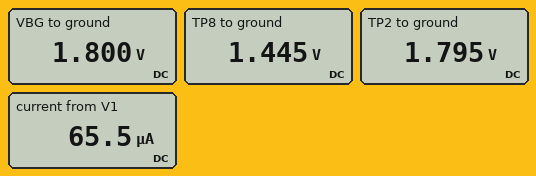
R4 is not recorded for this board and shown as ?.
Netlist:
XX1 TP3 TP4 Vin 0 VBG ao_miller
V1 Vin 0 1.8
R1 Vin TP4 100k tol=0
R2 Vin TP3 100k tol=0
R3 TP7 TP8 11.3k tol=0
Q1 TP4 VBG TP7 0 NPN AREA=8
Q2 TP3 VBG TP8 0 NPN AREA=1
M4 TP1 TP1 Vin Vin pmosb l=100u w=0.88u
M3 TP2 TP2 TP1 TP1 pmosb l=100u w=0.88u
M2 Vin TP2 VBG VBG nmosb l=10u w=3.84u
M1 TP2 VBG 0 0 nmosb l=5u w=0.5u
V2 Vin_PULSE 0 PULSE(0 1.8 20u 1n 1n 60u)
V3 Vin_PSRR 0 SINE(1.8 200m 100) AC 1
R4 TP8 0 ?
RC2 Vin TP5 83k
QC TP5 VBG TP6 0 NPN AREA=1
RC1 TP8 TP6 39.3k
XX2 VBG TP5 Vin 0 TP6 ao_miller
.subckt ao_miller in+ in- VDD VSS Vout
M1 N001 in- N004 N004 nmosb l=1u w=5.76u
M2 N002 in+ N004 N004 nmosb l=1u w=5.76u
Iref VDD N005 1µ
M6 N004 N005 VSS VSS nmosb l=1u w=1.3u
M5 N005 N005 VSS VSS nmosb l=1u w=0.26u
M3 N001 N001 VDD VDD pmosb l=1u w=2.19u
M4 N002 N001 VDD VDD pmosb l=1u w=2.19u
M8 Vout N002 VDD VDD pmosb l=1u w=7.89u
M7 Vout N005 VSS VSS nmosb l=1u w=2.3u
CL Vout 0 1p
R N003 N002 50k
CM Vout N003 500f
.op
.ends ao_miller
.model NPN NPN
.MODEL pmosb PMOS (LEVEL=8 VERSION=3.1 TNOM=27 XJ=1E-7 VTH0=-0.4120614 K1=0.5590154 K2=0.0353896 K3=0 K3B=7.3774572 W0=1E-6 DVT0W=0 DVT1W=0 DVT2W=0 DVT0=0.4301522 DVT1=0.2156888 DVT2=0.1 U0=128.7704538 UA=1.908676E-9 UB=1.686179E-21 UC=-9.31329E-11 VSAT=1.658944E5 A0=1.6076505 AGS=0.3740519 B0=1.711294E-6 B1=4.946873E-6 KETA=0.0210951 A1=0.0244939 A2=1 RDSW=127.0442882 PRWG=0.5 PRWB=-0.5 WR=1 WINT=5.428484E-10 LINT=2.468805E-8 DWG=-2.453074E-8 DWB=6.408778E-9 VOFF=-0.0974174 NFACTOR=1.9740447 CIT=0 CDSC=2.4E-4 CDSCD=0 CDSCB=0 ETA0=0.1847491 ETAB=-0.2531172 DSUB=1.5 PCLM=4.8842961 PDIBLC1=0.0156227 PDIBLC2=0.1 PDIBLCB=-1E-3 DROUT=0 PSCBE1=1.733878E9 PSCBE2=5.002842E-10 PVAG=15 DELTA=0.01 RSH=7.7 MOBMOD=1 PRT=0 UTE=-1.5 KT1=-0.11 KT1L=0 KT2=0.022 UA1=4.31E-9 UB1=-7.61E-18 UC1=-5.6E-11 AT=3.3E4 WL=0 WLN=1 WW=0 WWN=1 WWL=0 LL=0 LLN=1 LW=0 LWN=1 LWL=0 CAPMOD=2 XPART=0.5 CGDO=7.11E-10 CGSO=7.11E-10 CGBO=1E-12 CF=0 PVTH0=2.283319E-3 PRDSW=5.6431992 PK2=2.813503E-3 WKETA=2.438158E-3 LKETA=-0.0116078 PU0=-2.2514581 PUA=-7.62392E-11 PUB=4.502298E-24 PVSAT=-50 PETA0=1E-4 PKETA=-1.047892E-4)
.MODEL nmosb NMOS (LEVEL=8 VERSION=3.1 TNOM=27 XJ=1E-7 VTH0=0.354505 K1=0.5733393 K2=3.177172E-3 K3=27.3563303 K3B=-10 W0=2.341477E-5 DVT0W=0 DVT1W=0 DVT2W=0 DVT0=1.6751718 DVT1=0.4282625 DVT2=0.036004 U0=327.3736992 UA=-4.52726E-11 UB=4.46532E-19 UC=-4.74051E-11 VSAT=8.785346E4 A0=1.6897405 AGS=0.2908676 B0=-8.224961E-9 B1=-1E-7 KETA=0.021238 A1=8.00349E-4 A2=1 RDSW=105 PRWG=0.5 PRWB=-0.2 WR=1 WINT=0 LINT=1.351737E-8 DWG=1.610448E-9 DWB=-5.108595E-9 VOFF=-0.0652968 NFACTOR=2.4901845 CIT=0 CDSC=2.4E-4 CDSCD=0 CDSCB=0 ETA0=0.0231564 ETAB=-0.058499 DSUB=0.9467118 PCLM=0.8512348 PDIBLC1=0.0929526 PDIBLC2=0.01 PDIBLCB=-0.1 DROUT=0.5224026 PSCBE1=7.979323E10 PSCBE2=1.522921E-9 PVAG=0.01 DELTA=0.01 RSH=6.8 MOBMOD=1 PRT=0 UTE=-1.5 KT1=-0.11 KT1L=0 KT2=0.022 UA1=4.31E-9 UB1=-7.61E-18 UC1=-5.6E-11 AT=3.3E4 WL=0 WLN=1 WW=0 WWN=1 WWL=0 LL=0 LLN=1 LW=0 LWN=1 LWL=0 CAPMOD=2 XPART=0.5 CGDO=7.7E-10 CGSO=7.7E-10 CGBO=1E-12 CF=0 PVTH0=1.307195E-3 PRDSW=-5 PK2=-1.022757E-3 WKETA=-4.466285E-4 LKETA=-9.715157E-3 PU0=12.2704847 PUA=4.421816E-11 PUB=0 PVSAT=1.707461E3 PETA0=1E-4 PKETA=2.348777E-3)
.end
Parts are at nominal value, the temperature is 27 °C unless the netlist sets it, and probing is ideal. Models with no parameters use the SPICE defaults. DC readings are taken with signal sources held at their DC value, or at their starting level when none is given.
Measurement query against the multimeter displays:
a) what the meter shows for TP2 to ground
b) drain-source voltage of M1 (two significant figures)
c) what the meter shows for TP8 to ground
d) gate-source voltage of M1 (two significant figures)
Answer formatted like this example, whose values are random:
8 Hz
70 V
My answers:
1.795 V
1.8 V
1.445 V
1.8 V
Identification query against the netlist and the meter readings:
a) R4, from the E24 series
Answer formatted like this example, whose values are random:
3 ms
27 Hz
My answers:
160 kΩ
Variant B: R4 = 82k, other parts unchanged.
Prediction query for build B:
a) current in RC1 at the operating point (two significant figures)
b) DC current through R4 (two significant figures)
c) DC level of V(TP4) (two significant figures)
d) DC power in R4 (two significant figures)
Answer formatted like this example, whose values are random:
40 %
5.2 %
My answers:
14 µA
15 µA
1.7 V
19 µW
